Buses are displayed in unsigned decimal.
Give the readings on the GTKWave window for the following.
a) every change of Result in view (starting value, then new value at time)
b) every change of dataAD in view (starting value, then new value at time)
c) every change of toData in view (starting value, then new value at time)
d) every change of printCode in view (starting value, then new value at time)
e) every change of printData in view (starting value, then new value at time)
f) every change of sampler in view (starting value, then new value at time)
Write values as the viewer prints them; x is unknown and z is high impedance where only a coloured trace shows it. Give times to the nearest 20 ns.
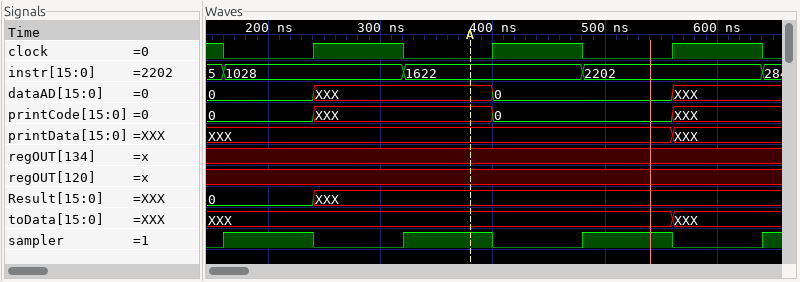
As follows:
0, XXX at 240 ns
0, XXX at 240 ns, 0 at 400 ns, XXX at 560 ns
XXX, XXX at 560 ns
0, XXX at 240 ns, 0 at 400 ns, XXX at 560 ns
XXX, XXX at 560 ns
0, 1 at 160 ns, 0 at 240 ns, 1 at 320 ns, 0 at 400 ns, 1 at 480 ns, 0 at 560 ns, 1 at 640 ns
